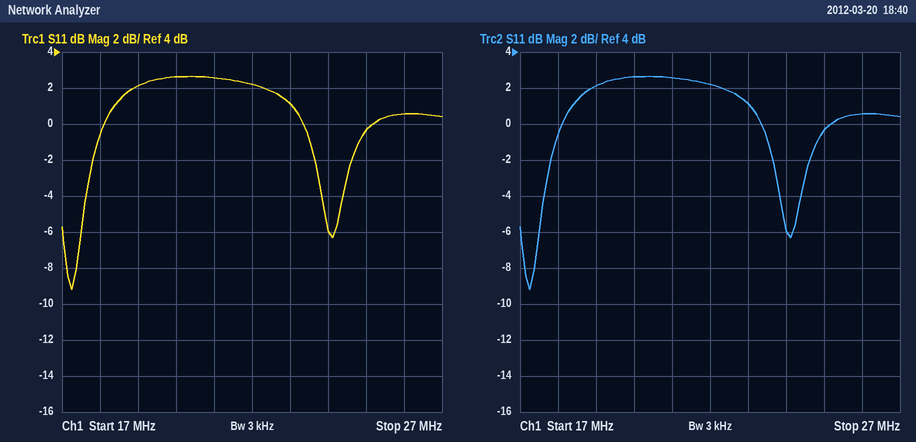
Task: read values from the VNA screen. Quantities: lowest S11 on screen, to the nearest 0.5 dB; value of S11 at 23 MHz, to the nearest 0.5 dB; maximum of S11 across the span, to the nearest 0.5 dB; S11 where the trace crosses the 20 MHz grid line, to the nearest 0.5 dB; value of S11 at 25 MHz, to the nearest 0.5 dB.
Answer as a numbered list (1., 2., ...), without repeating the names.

1. -9.0 dB
2. 1.0 dB
3. 2.5 dB
4. 2.5 dB
5. -0.5 dB
